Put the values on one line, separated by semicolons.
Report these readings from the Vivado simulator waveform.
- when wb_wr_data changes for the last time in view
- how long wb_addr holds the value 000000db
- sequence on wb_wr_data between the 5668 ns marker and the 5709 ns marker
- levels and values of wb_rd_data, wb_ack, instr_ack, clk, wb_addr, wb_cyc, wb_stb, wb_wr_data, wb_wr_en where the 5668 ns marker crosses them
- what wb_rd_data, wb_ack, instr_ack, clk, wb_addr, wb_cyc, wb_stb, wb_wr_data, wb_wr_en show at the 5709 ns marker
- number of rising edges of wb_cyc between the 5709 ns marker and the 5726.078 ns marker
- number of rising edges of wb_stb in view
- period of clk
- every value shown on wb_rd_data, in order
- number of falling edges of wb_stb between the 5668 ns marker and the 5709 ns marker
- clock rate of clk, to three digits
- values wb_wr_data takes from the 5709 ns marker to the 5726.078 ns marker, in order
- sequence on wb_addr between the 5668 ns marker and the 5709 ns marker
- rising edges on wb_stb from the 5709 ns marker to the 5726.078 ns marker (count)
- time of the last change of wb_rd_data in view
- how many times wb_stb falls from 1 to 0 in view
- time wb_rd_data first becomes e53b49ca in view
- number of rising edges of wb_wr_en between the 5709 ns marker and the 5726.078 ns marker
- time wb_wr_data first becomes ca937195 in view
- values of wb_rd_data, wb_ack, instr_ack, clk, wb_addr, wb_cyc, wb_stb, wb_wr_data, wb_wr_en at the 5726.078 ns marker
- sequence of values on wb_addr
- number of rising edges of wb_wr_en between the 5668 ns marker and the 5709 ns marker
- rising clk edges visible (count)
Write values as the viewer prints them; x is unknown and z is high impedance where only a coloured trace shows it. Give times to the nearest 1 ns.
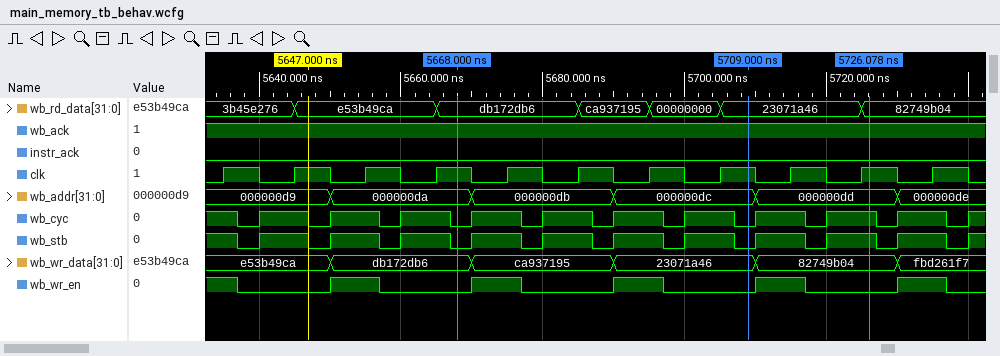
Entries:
5730 ns; 20 ns; db172db6, ca937195, 23071a46; wb_rd_data=db172db6, wb_ack=1, instr_ack=0, clk=1, wb_addr=000000da, wb_cyc=0, wb_stb=0, wb_wr_data=db172db6, wb_wr_en=0; wb_rd_data=23071a46, wb_ack=1, instr_ack=0, clk=1, wb_addr=000000dc, wb_cyc=0, wb_stb=0, wb_wr_data=23071a46, wb_wr_en=0; 2; 11; 10 ns; 3b45e276, e53b49ca, db172db6, ca937195, 00000000, 23071a46, 82749b04; 4; 100 MHz; 23071a46, 82749b04; 000000da, 000000db, 000000dc; 2; 5725 ns; 11; 5645 ns; 1; 5670 ns; wb_rd_data=82749b04, wb_ack=1, instr_ack=0, clk=1, wb_addr=000000dd, wb_cyc=1, wb_stb=1, wb_wr_data=82749b04, wb_wr_en=0; 000000d9, 000000da, 000000db, 000000dc, 000000dd, 000000de; 2; 11
